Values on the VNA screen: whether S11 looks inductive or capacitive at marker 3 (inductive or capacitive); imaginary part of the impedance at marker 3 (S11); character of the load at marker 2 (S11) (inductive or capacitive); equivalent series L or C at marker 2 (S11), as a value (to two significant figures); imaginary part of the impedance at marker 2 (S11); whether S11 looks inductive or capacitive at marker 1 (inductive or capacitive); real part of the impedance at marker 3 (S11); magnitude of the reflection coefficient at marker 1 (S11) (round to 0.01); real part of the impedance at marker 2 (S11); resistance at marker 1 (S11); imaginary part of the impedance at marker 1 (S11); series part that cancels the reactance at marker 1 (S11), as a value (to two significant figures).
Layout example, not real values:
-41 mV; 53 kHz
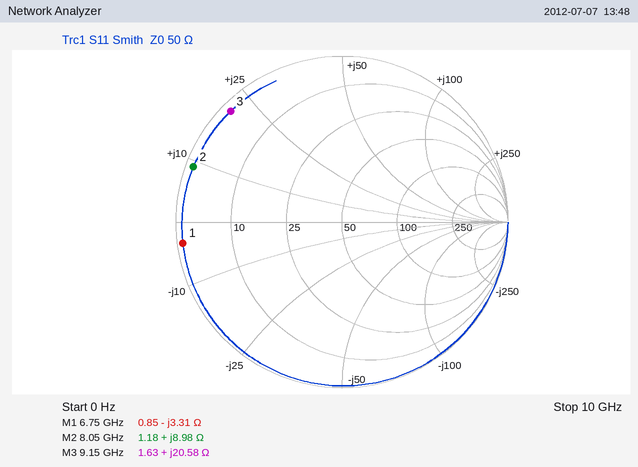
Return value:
inductive; +20.58 Ω; inductive; 180 pH; +8.98 Ω; capacitive; 1.63 Ω; 0.97; 1.18 Ω; 0.85 Ω; -3.31 Ω; 78 pH
